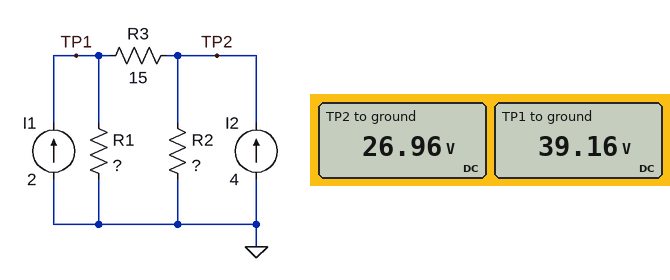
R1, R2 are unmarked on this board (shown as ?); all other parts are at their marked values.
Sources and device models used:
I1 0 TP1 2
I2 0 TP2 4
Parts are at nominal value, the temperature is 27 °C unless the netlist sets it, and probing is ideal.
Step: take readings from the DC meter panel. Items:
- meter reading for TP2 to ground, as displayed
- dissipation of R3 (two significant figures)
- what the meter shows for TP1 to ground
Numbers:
26.96 V
9.9 W
39.16 V
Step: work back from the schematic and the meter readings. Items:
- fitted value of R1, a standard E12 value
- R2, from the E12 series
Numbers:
33 Ω
5.6 Ω
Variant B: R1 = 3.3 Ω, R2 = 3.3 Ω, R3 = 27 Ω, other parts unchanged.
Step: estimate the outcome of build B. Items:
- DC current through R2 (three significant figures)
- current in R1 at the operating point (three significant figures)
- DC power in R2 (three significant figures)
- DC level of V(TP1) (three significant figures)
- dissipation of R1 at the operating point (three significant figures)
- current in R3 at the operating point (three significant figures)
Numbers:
3.80 A
2.20 A
47.7 W
7.25 V
15.9 W
196 mA
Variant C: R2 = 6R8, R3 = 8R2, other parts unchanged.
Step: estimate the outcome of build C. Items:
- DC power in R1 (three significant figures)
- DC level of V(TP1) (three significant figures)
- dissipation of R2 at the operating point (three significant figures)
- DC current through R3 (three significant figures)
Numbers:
46.9 W
39.3 V
157 W
808 mA
